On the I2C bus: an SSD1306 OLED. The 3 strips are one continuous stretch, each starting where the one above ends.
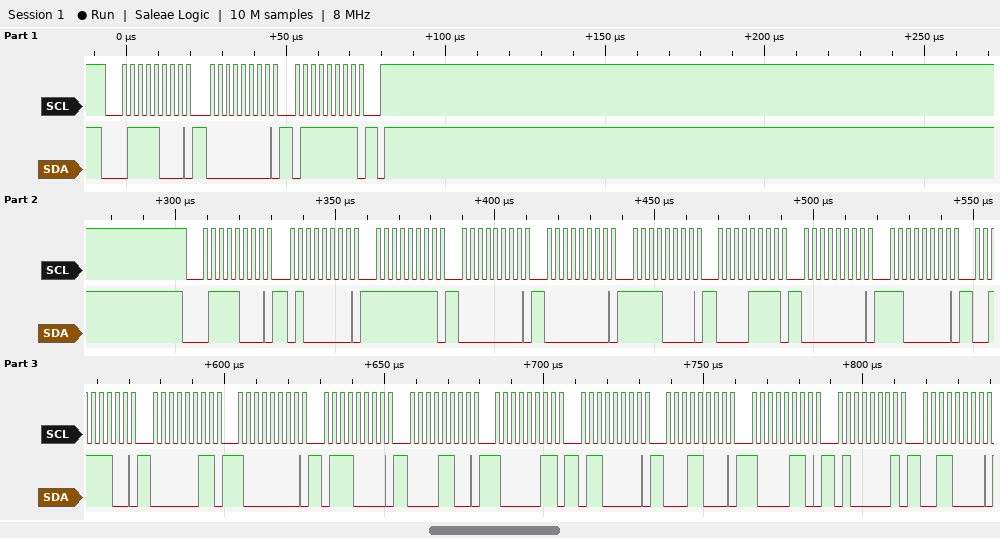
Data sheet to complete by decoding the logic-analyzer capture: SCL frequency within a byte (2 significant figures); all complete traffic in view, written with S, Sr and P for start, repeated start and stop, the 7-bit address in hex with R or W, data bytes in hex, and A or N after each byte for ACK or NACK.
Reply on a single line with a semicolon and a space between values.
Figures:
400 kHz; S 3CW A 00 A 7F A P S 3CW A 40 A FF A 00 A 00 A F0 A 0F A 00 A C0 A 3C A 03 A 80 A 70 A 0C A 83 A 60 A 18 A 86 A 41 A 30 A
